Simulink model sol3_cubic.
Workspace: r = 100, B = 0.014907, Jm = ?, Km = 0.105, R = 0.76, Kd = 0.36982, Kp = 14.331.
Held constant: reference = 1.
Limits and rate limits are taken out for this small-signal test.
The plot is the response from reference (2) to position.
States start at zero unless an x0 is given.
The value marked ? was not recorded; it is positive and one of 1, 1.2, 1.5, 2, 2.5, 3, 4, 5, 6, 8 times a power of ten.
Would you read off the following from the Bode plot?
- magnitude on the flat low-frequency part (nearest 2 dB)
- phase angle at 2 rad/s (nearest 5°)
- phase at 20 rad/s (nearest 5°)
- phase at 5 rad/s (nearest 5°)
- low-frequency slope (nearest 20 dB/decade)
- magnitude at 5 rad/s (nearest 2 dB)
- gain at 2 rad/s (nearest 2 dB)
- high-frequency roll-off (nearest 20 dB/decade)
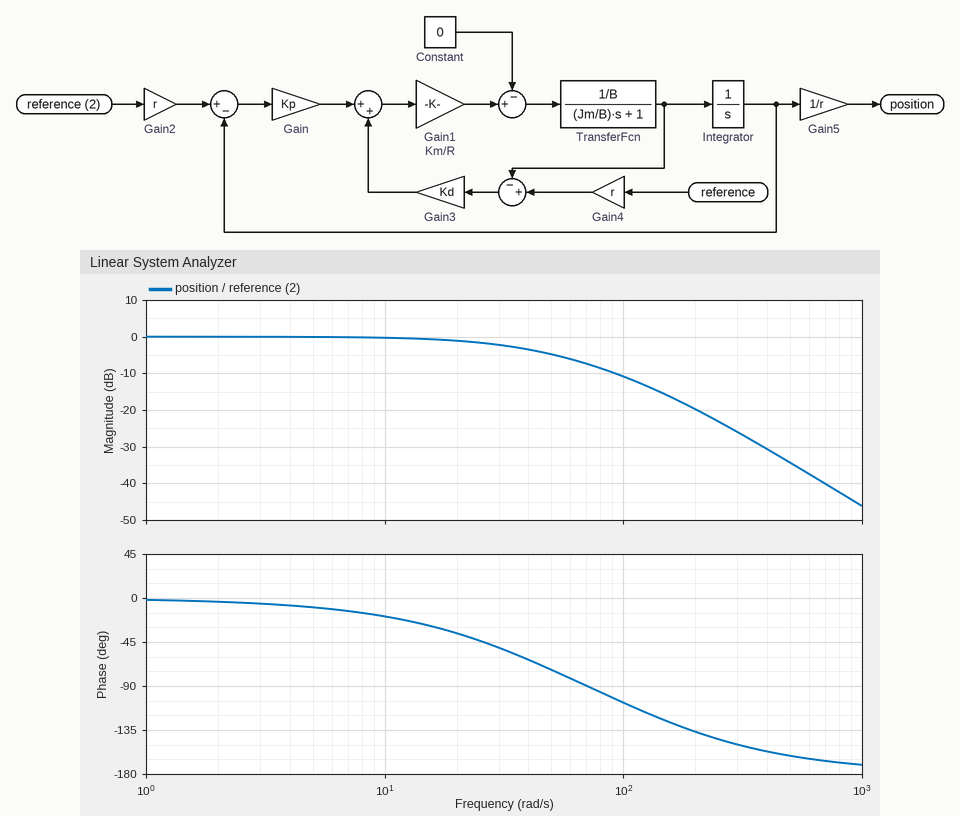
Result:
0 dB
-5°
-35°
-10°
0 dB/decade
0 dB
0 dB
-40 dB/decade
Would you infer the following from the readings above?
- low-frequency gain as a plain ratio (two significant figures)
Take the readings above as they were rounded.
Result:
1.0
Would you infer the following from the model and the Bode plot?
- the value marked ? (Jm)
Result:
0.0004
